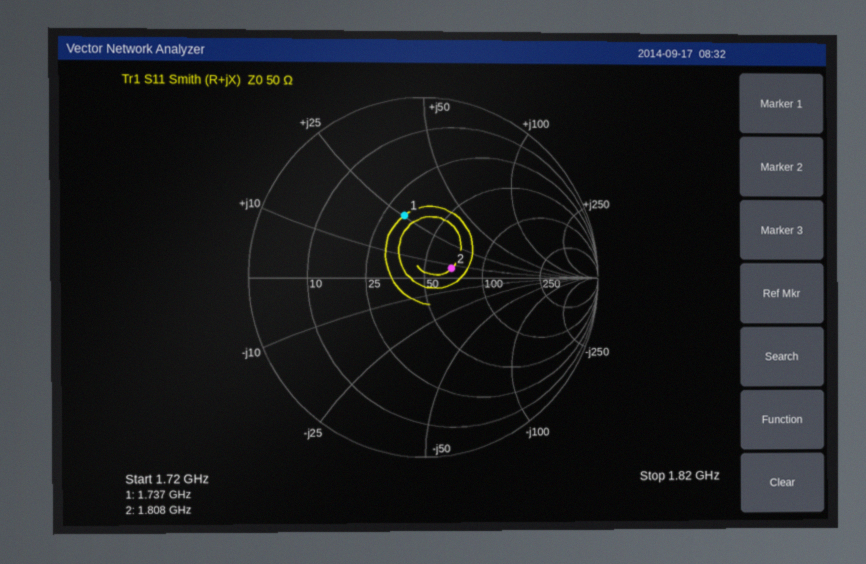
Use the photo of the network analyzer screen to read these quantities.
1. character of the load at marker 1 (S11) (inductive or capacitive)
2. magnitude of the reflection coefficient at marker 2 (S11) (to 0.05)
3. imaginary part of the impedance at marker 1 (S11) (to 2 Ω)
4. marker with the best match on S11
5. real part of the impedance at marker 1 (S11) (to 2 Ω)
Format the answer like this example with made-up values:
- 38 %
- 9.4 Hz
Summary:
- inductive
- 0.15
- +26 Ω
- marker 2
- 32 Ω
